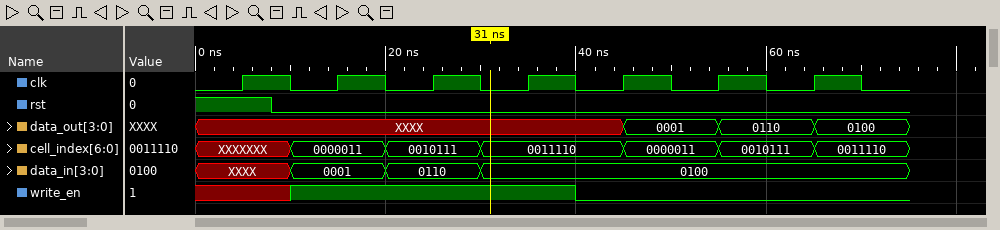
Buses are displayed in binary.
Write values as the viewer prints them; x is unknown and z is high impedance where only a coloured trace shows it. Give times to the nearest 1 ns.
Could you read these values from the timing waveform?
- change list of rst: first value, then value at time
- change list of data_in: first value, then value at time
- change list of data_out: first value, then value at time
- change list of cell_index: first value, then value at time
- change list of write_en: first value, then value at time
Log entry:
1, 0 at 8 ns
XXXX, 0001 at 10 ns, 0110 at 20 ns, 0100 at 30 ns
XXXX, 0001 at 45 ns, 0110 at 55 ns, 0100 at 65 ns
XXXXXXX, 0000011 at 10 ns, 0010111 at 20 ns, 0011110 at 30 ns, 0000011 at 45 ns, 0010111 at 55 ns, 0011110 at 65 ns
x, 1 at 10 ns, 0 at 40 ns
